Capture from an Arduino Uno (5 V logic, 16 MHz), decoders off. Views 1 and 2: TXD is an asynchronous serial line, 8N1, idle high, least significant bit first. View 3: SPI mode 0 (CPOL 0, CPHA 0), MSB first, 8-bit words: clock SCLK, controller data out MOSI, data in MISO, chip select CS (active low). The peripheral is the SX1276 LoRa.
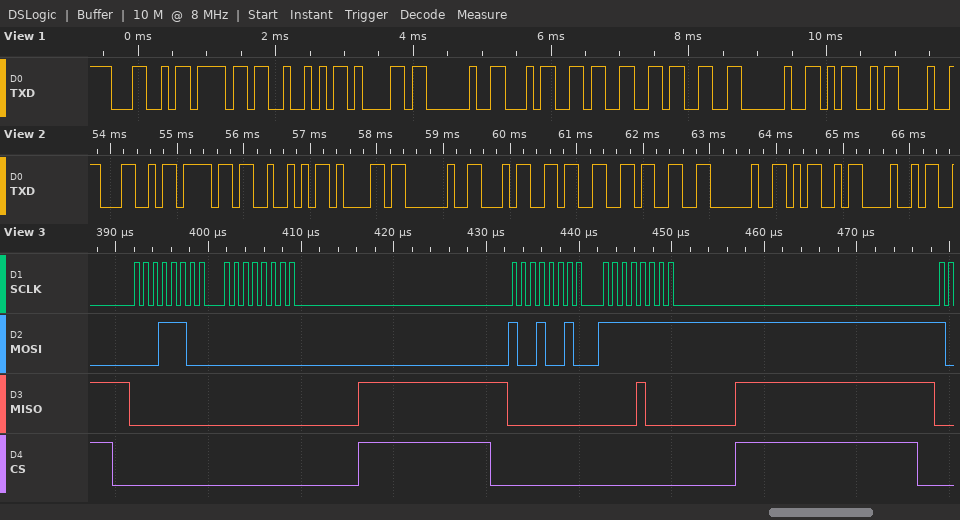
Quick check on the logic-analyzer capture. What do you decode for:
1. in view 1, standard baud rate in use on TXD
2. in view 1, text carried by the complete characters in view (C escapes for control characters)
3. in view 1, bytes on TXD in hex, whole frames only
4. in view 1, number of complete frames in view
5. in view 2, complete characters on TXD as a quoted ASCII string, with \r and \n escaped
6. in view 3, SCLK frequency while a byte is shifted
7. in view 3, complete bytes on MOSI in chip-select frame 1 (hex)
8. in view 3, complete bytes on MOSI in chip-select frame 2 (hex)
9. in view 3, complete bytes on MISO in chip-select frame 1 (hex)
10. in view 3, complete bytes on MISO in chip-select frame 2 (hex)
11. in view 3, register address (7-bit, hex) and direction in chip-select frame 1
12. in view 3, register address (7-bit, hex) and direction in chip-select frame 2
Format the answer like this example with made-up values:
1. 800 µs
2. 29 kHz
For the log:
1. 9600 baud
2. "LoRa 433 M"
3. 4C 6F 52 61 20 34 33 33 20 4D
4. 10
5. "LoRa 433 MH"
6. 1 MHz
7. 1C 00
8. 92 FF
9. 00 00
10. 00 08
11. 0x1C read
12. 0x12 write
